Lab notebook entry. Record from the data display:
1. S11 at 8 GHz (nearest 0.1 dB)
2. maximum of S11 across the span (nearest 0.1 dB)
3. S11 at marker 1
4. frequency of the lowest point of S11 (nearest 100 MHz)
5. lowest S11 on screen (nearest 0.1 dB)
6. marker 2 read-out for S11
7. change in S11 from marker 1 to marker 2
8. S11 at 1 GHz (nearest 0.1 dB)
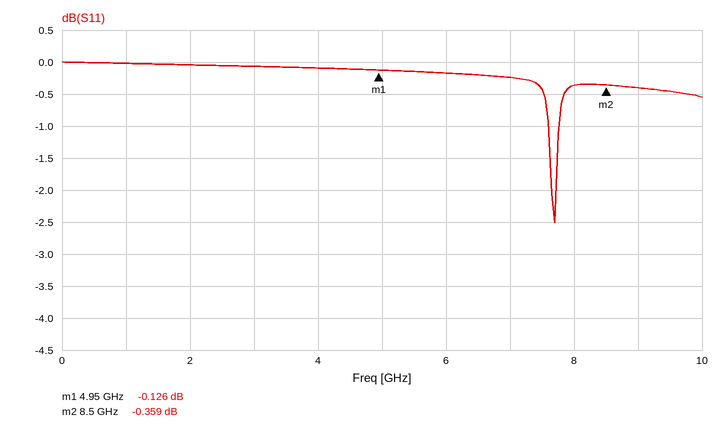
-0.4 dB
0.0 dB
-0.126 dB
7.7 GHz
-2.5 dB
-0.359 dB
-0.233 dB
0.0 dB
